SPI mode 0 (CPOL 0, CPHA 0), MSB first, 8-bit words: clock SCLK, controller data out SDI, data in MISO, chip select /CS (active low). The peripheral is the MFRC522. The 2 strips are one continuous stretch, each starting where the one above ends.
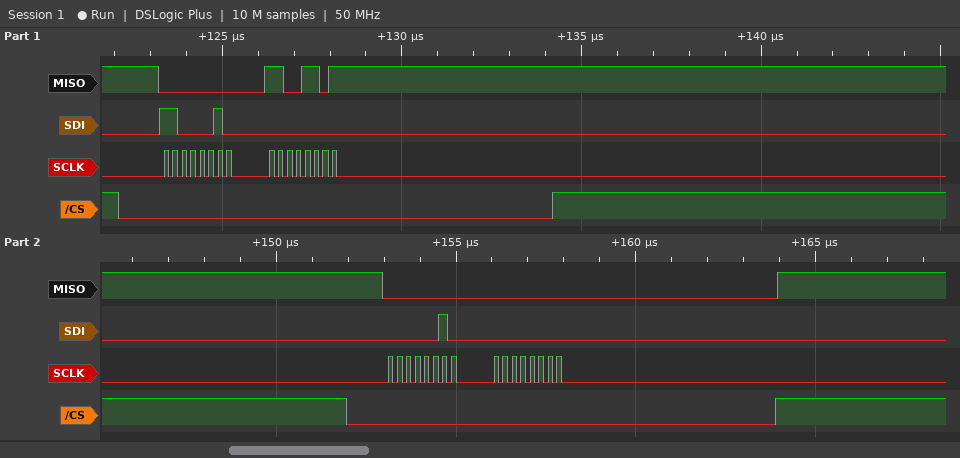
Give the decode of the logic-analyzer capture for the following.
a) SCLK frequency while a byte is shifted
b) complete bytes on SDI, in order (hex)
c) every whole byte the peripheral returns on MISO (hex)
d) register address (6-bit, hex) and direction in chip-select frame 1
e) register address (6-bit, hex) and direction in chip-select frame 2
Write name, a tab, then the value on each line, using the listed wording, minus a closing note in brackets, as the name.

SCLK frequency while a byte is shifted	4 MHz
complete bytes on SDI, in order	C2 00 02 00
every whole byte the peripheral returns on MISO	00 CD 00 00
register address (6-bit, hex) and direction in chip-select frame 1	0x21 read
register address (6-bit, hex) and direction in chip-select frame 2	0x01 write
